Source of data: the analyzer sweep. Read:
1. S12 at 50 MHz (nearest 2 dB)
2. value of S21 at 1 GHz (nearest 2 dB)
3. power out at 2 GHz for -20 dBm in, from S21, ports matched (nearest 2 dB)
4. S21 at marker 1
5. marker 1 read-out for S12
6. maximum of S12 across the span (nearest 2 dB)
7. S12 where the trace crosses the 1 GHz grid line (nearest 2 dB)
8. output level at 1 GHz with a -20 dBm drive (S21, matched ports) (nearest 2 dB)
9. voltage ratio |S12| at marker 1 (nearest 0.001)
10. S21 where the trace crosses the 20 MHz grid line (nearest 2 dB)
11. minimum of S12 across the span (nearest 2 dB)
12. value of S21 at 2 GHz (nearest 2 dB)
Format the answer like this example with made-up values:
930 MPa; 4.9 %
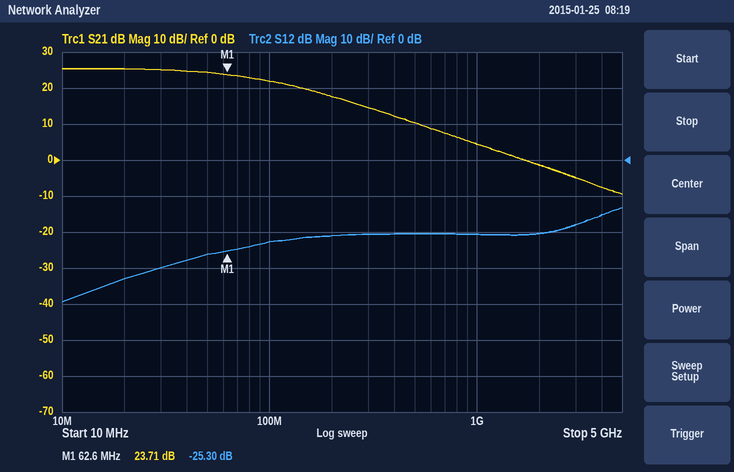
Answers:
-26 dB; 4 dB; -22 dBm; 23.71 dB; -25.30 dB; -14 dB; -20 dB; -16 dBm; 0.054; 26 dB; -40 dB; -2 dB
